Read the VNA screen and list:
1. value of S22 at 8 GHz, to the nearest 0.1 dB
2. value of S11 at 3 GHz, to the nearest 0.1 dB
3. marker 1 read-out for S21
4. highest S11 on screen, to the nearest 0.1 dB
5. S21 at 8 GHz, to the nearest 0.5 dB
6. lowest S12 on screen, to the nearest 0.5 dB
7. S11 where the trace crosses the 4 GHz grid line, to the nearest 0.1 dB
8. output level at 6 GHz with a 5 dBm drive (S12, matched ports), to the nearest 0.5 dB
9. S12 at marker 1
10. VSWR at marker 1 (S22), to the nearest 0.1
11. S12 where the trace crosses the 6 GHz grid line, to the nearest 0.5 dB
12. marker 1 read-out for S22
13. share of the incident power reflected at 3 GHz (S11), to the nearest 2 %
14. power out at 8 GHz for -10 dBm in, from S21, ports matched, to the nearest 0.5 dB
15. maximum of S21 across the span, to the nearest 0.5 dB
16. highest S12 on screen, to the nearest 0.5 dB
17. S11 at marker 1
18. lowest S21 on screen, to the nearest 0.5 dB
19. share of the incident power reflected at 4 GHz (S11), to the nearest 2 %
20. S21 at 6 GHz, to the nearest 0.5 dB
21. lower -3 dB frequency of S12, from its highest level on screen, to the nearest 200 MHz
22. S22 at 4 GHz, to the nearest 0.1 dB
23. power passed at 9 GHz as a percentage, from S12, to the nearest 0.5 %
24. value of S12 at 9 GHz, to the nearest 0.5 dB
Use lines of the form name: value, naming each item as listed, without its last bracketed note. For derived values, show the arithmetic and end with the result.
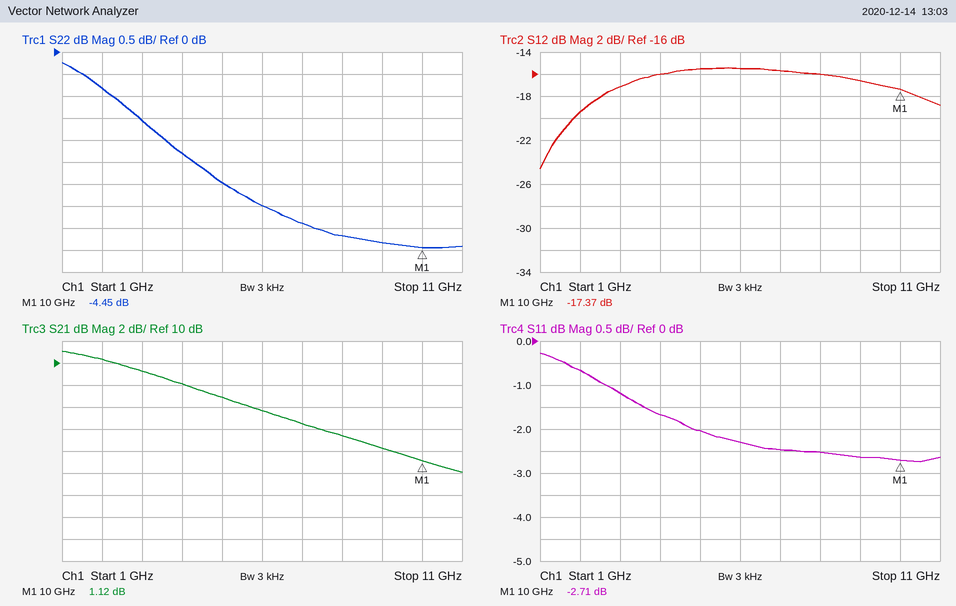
value of S22 at 8 GHz, to the nearest 0.1 dB: -4.2 dB
value of S11 at 3 GHz, to the nearest 0.1 dB: -1.2 dB
marker 1 read-out for S21: 1.12 dB
highest S11 on screen, to the nearest 0.1 dB: -0.3 dB
S21 at 8 GHz, to the nearest 0.5 dB: 3.5 dB
lowest S12 on screen, to the nearest 0.5 dB: -24.5 dB
S11 where the trace crosses the 4 GHz grid line, to the nearest 0.1 dB: -1.7 dB
output level at 6 GHz with a 5 dBm drive (S12, matched ports), to the nearest 0.5 dB: 5 dBm + (-15.5 dB) = -10.5 dBm
S12 at marker 1: -17.37 dB
VSWR at marker 1 (S22), to the nearest 0.1: (1 + 0.5991)/(1 − 0.5991) ≈ 4.0
S12 where the trace crosses the 6 GHz grid line, to the nearest 0.5 dB: -15.5 dB
marker 1 read-out for S22: -4.45 dB
share of the incident power reflected at 3 GHz (S11), to the nearest 2 %: 10^(-1.2/10) ≈ 76 %
power out at 8 GHz for -10 dBm in, from S21, ports matched, to the nearest 0.5 dB: -10 dBm + (3.5 dB) = -6.5 dBm
maximum of S21 across the span, to the nearest 0.5 dB: 11.0 dB
highest S12 on screen, to the nearest 0.5 dB: -15.5 dB
S11 at marker 1: -2.71 dB
lowest S21 on screen, to the nearest 0.5 dB: 0.0 dB
share of the incident power reflected at 4 GHz (S11), to the nearest 2 %: 10^(-1.7/10) ≈ 68 %
S21 at 6 GHz, to the nearest 0.5 dB: 5.5 dB
lower -3 dB frequency of S12, from its highest level on screen, to the nearest 200 MHz: 2.4 GHz
S22 at 4 GHz, to the nearest 0.1 dB: -2.3 dB
power passed at 9 GHz as a percentage, from S12, to the nearest 0.5 %: 10^(-16.5/10) ≈ 2.24 %, so 2.0 % to the nearest 0.5 %
value of S12 at 9 GHz, to the nearest 0.5 dB: -16.5 dB
